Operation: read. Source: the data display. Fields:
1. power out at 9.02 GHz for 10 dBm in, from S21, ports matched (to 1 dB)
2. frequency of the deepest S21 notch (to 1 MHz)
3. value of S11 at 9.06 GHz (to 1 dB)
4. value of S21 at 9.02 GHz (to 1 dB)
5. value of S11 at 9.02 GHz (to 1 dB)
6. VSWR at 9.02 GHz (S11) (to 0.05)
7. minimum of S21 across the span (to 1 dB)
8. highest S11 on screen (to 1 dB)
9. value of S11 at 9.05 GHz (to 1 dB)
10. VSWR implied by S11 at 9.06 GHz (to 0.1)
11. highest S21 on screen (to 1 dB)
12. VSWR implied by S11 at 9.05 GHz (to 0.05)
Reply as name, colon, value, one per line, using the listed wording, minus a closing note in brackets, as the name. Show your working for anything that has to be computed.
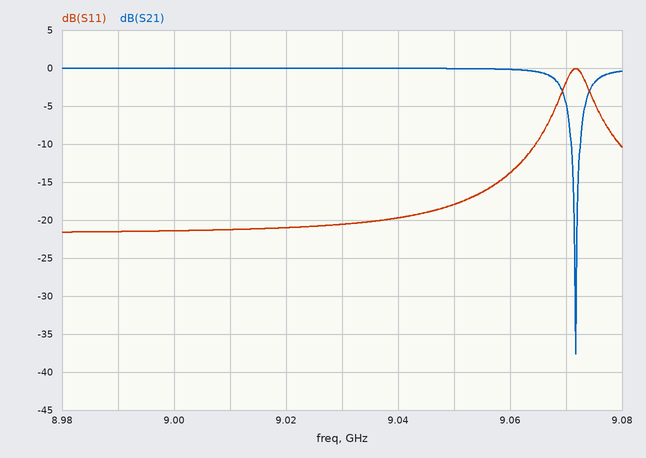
power out at 9.02 GHz for 10 dBm in, from S21, ports matched: 10 dBm + (0 dB) = 10 dBm
frequency of the deepest S21 notch: 9.072 GHz
value of S11 at 9.06 GHz: -14 dB
value of S21 at 9.02 GHz: 0 dB
value of S11 at 9.02 GHz: -21 dB
VSWR at 9.02 GHz (S11): |Γ| = 10^(-21/20) = 0.0891; VSWR = (1 + 0.0891)/(1 − 0.0891) ≈ 1.20
minimum of S21 across the span: -38 dB
highest S11 on screen: 0 dB
value of S11 at 9.05 GHz: -18 dB
VSWR implied by S11 at 9.06 GHz: |Γ| = 10^(-14/20) = 0.1995; VSWR = (1 + 0.1995)/(1 − 0.1995) ≈ 1.5
highest S21 on screen: 0 dB
VSWR implied by S11 at 9.05 GHz: |Γ| = 10^(-18/20) = 0.1259; VSWR = (1 + 0.1259)/(1 − 0.1259) ≈ 1.29, so 1.30 to the nearest 0.05
